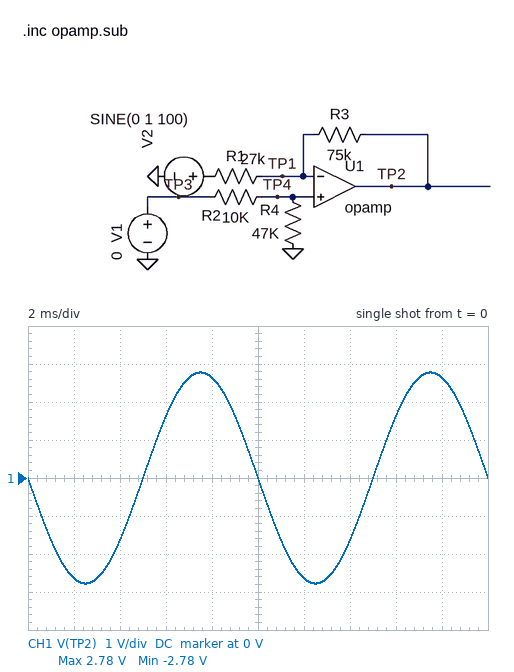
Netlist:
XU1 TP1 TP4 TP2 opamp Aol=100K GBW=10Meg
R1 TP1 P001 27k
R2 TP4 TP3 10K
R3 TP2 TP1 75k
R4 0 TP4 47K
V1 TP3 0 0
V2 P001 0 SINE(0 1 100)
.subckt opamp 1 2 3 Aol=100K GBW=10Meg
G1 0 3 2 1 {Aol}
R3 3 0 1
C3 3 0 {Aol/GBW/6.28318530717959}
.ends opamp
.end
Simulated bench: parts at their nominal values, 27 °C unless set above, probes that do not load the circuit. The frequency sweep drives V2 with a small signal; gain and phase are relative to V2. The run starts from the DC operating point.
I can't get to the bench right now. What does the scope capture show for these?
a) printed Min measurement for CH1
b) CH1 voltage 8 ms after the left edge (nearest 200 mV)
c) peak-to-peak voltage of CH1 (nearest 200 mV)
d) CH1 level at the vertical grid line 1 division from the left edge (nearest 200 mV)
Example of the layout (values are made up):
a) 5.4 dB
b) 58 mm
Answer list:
a) -2.78 V
b) 2.6 V
c) 5.6 V
d) -2.6 V
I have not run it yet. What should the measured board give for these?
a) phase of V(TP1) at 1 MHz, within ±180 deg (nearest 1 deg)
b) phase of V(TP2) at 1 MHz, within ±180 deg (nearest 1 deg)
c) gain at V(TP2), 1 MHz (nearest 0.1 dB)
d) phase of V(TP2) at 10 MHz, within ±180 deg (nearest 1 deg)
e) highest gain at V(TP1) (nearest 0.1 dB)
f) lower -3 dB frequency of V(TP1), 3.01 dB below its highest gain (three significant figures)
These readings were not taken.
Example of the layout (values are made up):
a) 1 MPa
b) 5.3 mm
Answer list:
a) 69 deg
b) 159 deg
c) 8.3 dB
d) 105 deg
e) -2.7 dB
f) 2.65 MHz
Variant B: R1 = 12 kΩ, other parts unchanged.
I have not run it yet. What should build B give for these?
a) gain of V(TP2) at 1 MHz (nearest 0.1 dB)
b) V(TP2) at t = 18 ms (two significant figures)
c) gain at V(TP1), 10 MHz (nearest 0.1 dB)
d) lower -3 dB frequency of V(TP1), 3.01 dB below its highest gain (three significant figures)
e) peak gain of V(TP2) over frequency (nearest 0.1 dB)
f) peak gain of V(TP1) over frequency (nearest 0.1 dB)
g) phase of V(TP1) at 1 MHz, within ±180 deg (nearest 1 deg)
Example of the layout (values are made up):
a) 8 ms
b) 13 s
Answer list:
a) 14.1 dB
b) 5.9 V
c) -1.4 dB
d) 1.38 MHz
e) 15.9 dB
f) -1.3 dB
g) 54 deg
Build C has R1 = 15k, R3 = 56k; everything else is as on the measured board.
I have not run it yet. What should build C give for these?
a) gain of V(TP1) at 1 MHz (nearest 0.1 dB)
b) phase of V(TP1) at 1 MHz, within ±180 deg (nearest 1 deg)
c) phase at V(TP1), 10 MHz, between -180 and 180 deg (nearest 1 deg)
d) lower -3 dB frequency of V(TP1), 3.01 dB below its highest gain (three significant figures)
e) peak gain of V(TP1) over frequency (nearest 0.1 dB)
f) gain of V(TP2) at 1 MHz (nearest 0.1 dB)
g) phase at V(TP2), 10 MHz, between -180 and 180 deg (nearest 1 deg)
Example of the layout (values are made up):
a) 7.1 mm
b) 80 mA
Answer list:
a) -9.4 dB
b) 65 deg
c) 12 deg
d) 2.11 MHz
e) -2.1 dB
f) 10.6 dB
g) 102 deg
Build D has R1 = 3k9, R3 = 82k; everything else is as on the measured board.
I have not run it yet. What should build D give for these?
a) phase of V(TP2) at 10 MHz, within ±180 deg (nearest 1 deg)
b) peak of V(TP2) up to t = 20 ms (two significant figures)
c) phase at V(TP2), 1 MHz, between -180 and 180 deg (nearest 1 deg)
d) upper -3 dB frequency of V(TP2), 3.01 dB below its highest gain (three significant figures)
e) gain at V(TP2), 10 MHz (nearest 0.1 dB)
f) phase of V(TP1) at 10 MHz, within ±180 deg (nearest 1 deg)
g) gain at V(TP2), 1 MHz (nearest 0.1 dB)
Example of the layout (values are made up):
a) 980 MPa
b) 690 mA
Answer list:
a) 93 deg
b) 21 V
c) 114 deg
d) 454 kHz
e) -0.4 dB
f) 3 deg
g) 18.8 dB
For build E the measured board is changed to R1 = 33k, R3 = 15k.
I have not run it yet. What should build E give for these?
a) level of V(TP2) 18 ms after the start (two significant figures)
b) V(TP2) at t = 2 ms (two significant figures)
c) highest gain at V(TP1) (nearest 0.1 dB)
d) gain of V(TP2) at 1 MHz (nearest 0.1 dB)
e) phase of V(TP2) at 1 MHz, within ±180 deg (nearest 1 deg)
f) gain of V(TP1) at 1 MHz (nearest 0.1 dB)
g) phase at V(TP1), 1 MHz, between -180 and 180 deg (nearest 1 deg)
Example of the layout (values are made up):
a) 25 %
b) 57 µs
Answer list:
a) 430 mV
b) -430 mV
c) -10.1 dB
d) -6.9 dB
e) 172 deg
f) -26.9 dB
g) 82 deg
